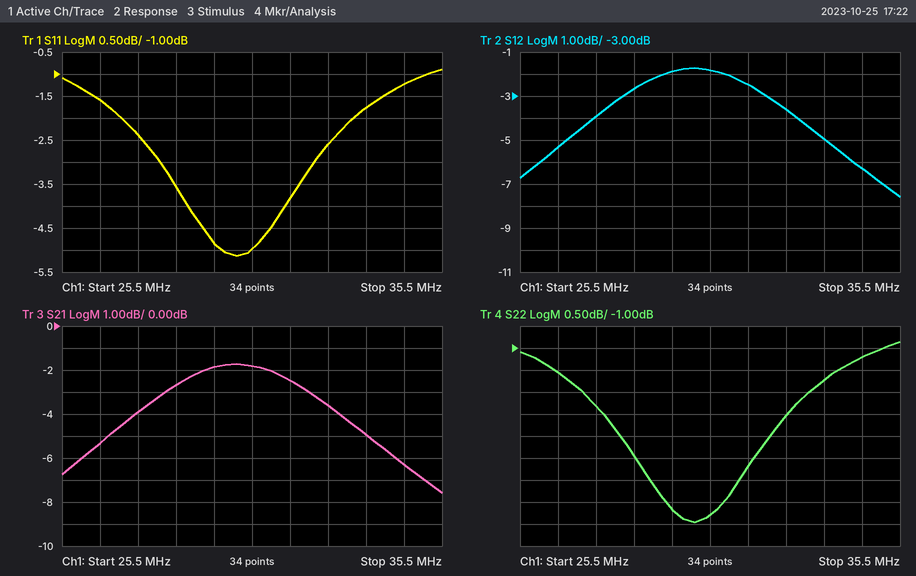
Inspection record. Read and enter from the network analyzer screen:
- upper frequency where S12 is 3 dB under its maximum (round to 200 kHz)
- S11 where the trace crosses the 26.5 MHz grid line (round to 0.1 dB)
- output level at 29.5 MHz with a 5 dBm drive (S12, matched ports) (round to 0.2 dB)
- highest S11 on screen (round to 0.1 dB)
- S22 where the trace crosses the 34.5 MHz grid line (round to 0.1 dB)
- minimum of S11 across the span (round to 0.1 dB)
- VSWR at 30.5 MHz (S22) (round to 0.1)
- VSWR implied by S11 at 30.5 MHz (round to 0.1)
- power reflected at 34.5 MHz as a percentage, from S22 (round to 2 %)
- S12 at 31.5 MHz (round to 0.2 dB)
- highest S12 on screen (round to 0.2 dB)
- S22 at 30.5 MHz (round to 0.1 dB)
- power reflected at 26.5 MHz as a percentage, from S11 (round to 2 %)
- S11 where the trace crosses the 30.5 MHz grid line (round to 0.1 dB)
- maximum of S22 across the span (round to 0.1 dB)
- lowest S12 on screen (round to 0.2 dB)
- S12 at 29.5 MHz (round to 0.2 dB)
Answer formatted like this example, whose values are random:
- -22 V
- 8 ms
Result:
- 33.4 MHz
- -1.6 dB
- 3.2 dBm
- -0.9 dB
- -1.2 dB
- -5.1 dB
- 3.7
- 3.6
- 76 %
- -2.4 dB
- -1.8 dB
- -4.8 dB
- 70 %
- -5.0 dB
- -0.9 dB
- -7.6 dB
- -1.8 dB
